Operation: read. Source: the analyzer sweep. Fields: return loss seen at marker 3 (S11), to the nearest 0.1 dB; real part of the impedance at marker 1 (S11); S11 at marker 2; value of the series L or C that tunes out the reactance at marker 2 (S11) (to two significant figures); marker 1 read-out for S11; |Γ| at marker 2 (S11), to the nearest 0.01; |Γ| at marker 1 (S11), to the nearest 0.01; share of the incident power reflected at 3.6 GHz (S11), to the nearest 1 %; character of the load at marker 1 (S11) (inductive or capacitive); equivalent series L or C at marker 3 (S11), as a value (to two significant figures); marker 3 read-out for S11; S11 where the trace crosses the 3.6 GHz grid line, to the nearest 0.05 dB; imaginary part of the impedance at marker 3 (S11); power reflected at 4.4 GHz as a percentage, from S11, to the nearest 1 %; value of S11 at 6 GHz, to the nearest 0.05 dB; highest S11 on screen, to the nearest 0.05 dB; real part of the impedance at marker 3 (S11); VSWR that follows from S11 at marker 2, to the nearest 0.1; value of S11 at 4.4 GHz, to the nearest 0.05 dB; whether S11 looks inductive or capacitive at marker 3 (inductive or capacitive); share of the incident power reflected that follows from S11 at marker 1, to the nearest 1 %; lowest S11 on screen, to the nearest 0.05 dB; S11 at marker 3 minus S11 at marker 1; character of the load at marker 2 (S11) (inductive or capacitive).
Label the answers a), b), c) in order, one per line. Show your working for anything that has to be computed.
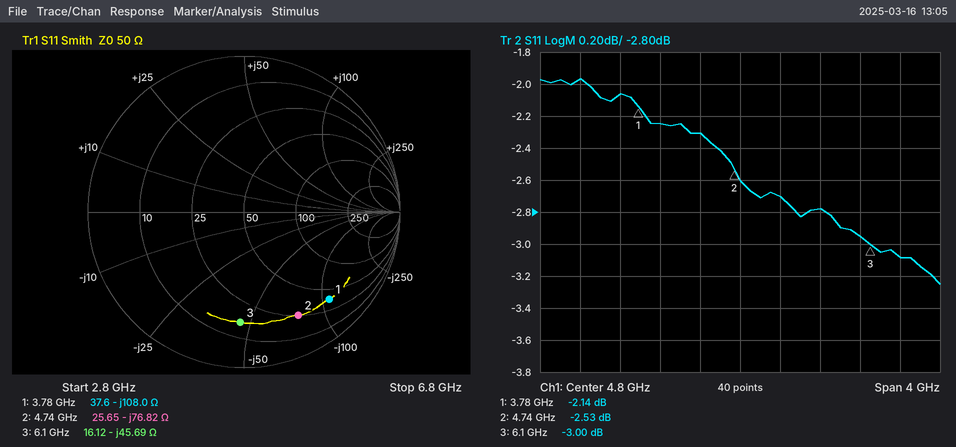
a) 3.0 dB
b) 37.6 Ω
c) -2.53 dB
d) L = 76.82 Ω/(2π × 4.74 GHz) ≈ 2.6 nH
e) -2.14 dB
f) 0.75
g) 0.78
h) 10^(-2.05/10) ≈ 62 %
i) capacitive
j) C = 1/(2π × 6.1 GHz × 45.69 Ω) ≈ 571 fF, so 570 fF to two significant figures
k) -3.00 dB
l) -2.05 dB
m) -45.69 Ω
n) 10^(-2.3/10) ≈ 59 %
o) -2.95 dB
p) -1.95 dB
q) 16.12 Ω
r) (1 + 0.7473)/(1 − 0.7473) ≈ 6.9
s) -2.30 dB
t) capacitive
u) 10^(-2.14/10) ≈ 61 %
v) -3.25 dB
w) -3 − (-2.14) = -0.86 dB
x) capacitive
